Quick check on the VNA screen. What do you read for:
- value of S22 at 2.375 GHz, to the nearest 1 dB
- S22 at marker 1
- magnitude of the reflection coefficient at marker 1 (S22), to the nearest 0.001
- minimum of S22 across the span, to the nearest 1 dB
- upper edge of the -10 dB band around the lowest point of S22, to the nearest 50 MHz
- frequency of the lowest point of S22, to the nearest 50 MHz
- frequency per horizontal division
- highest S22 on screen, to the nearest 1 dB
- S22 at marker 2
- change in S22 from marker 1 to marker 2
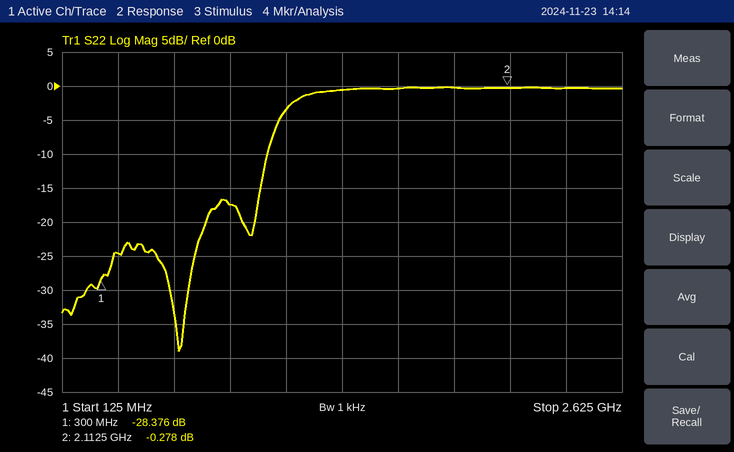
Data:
0 dB
-28.376 dB
0.038
-39 dB
1.05 GHz
650 MHz
250 MHz
0 dB
-0.278 dB
28.098 dB
